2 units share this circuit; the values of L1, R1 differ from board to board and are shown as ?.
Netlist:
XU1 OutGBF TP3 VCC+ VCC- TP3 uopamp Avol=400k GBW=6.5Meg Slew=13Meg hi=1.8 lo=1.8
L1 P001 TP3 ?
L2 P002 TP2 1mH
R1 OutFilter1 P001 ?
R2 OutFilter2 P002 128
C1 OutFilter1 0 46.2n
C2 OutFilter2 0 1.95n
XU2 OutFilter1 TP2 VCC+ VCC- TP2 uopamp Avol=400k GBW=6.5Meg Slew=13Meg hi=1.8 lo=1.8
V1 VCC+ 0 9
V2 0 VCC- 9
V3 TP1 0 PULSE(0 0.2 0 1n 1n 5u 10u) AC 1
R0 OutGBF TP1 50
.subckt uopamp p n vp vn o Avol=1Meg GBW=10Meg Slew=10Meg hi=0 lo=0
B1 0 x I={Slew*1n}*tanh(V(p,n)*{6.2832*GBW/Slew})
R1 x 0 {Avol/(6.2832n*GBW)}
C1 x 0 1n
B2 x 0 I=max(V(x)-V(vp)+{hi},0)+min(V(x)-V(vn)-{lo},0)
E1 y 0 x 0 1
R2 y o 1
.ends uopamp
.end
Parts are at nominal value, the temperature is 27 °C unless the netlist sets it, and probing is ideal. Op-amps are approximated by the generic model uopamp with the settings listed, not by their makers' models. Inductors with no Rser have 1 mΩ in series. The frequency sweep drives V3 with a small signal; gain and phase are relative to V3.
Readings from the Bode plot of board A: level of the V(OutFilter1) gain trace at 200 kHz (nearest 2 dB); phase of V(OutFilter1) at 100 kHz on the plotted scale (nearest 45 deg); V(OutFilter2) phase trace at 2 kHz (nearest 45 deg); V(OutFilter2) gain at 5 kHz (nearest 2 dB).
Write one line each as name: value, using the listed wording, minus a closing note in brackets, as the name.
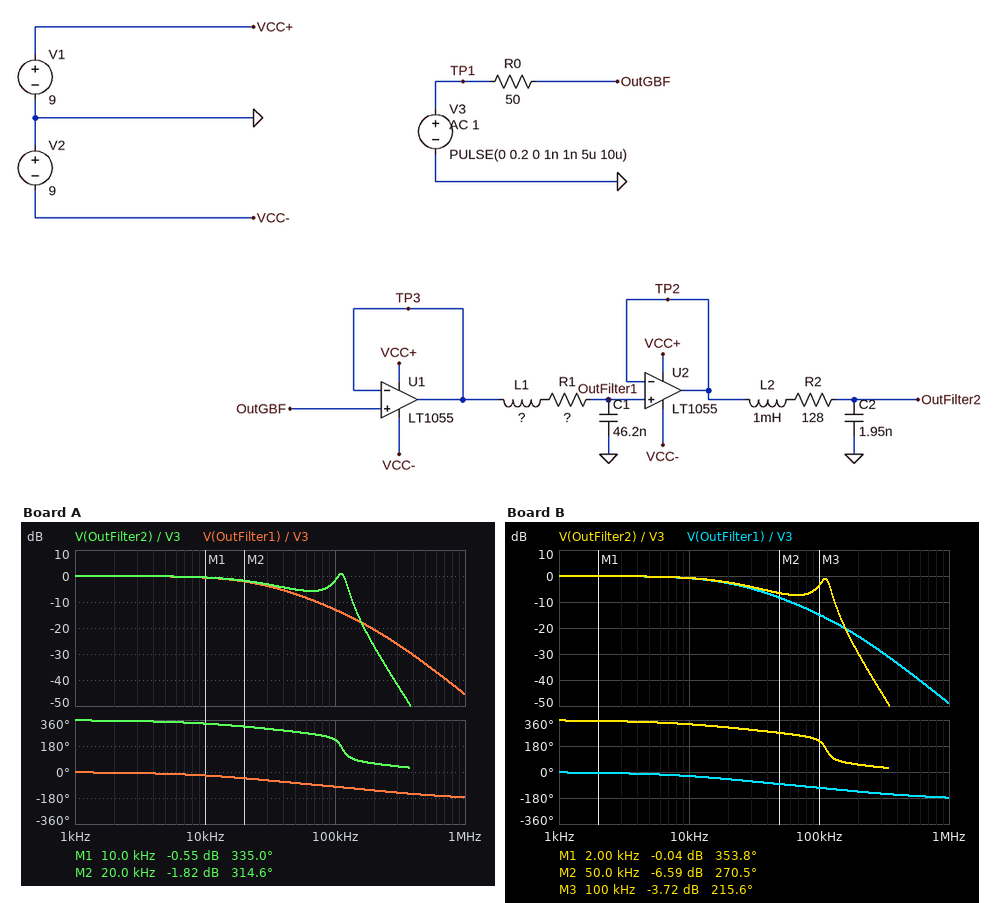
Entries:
level of the V(OutFilter1) gain trace at 200 kHz: -20 dB
phase of V(OutFilter1) at 100 kHz on the plotted scale: -90 deg
V(OutFilter2) phase trace at 2 kHz: 360 deg
V(OutFilter2) gain at 5 kHz: 0 dB
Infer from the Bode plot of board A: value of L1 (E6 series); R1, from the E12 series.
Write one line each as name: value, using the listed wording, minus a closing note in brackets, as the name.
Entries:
value of L1: 100 µH
R1, from the E12 series: 150 Ω
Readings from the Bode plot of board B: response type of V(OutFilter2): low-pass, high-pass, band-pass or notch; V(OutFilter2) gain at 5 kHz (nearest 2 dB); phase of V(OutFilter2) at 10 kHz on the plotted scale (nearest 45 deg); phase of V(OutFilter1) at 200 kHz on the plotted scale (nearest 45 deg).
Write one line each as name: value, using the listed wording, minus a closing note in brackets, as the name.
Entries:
response type of V(OutFilter2): low-pass, high-pass, band-pass or notch: low-pass
V(OutFilter2) gain at 5 kHz: 0 dB
phase of V(OutFilter2) at 10 kHz on the plotted scale: 315 deg
phase of V(OutFilter1) at 200 kHz on the plotted scale: -135 deg
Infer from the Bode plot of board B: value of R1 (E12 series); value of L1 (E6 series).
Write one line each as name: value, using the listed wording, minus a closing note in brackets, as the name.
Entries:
value of R1: 180 Ω
value of L1: 150 µH
